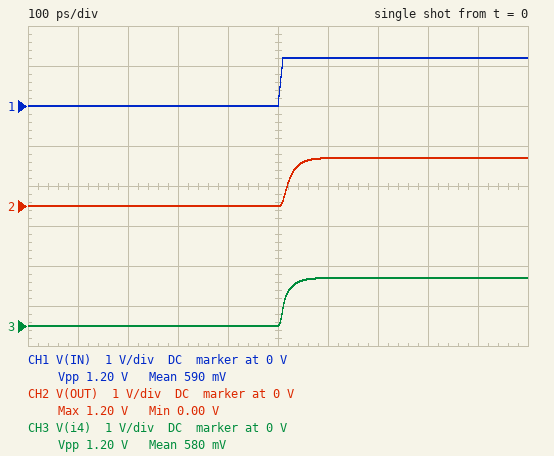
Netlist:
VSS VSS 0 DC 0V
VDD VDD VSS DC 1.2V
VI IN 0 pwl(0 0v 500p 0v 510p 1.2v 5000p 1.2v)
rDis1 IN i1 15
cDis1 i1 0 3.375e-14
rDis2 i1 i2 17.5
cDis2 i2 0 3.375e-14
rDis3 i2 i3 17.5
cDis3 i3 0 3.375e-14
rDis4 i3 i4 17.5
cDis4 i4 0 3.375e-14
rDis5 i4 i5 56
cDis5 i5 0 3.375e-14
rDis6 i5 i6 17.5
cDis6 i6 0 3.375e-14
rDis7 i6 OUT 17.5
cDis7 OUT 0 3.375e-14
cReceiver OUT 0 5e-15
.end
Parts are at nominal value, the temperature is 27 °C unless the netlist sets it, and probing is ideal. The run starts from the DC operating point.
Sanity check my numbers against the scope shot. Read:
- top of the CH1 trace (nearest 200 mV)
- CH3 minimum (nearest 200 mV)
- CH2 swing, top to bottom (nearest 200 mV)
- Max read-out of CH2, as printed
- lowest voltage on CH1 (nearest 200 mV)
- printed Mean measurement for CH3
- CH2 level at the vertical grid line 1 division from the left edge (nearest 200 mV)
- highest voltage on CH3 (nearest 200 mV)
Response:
1.2 V
0 V
1.2 V
1.20 V
0 V
580 mV
0 V
1.2 V
